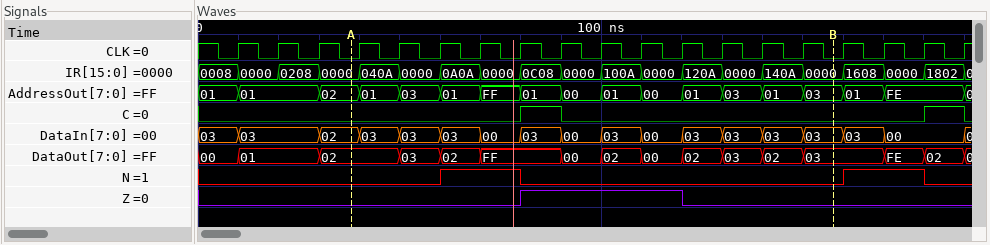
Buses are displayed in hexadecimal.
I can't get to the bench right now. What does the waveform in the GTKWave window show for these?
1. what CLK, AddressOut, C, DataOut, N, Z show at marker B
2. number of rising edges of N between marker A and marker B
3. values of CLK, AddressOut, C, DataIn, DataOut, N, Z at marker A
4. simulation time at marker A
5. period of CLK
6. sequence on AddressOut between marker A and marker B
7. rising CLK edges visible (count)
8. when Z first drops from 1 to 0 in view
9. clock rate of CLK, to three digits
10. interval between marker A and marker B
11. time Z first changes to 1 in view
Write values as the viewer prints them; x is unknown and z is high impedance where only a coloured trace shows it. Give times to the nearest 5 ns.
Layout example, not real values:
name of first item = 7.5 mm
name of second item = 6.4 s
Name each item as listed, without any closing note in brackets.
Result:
what CLK, AddressOut, C, DataOut, N, Z show at marker B = CLK=0, AddressOut=03, C=0, DataOut=03, N=0, Z=0
number of rising edges of N between marker A and marker B = 1
values of CLK, AddressOut, C, DataIn, DataOut, N, Z at marker A = CLK=0, AddressOut=02, C=0, DataIn=02, DataOut=02, N=0, Z=0
simulation time at marker A = 40 ns
period of CLK = 10 ns
sequence on AddressOut between marker A and marker B = 02, 01, 03, 01, FF, 01, 00, 01, 00, 01, 03, 01, 03
rising CLK edges visible = 19
when Z first drops from 1 to 0 in view = 120 ns
clock rate of CLK, to three digits = 100 MHz
interval between marker A and marker B = 120 ns
time Z first changes to 1 in view = 80 ns
